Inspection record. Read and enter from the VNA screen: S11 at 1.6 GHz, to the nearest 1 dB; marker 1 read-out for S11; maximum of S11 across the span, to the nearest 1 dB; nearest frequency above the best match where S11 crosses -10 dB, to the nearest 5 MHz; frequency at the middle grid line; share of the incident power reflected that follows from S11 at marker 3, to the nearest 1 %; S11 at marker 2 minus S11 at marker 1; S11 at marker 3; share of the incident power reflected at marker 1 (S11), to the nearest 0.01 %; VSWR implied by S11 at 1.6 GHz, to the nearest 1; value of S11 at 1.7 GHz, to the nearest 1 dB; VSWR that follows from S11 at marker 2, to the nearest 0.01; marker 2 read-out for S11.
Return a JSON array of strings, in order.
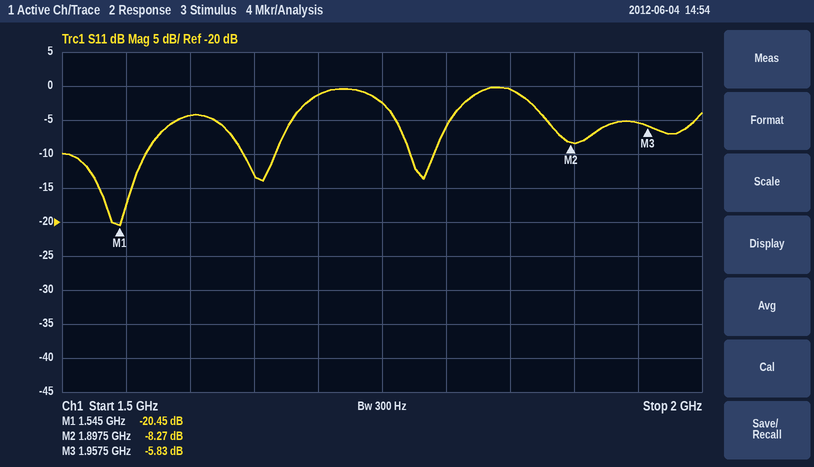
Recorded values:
["-4 dB", "-20.45 dB", "0 dB", "1.565 GHz", "1.75 GHz", "26 %", "12.18 dB", "-5.83 dB", "0.90 %", "4", "-1 dB", "2.26", "-8.27 dB"]
